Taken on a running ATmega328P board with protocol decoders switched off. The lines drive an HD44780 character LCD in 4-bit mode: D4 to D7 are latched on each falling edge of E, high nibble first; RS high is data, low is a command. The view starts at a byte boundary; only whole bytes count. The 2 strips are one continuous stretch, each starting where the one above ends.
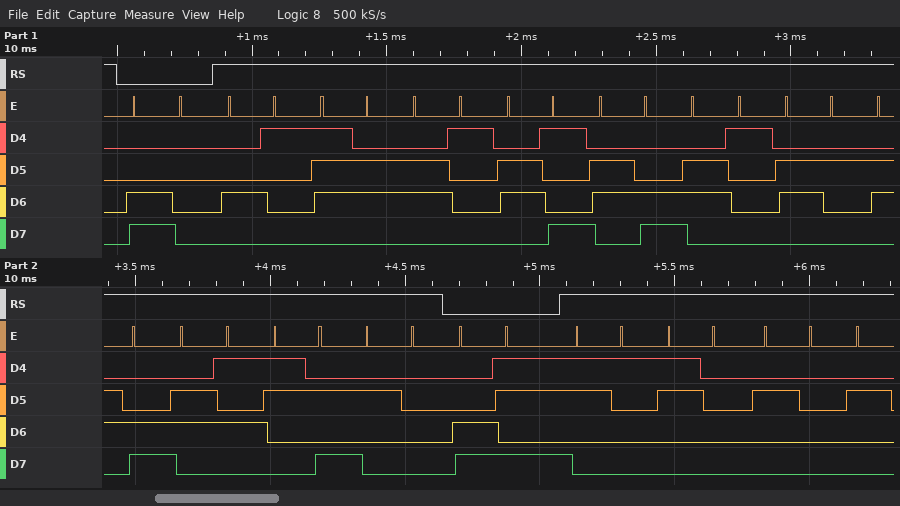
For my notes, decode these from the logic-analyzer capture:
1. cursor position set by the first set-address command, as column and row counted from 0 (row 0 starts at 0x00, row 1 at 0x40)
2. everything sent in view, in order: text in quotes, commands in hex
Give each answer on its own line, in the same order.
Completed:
column 0, row 1
0xC0 "Available: " 0xCB "10 "
